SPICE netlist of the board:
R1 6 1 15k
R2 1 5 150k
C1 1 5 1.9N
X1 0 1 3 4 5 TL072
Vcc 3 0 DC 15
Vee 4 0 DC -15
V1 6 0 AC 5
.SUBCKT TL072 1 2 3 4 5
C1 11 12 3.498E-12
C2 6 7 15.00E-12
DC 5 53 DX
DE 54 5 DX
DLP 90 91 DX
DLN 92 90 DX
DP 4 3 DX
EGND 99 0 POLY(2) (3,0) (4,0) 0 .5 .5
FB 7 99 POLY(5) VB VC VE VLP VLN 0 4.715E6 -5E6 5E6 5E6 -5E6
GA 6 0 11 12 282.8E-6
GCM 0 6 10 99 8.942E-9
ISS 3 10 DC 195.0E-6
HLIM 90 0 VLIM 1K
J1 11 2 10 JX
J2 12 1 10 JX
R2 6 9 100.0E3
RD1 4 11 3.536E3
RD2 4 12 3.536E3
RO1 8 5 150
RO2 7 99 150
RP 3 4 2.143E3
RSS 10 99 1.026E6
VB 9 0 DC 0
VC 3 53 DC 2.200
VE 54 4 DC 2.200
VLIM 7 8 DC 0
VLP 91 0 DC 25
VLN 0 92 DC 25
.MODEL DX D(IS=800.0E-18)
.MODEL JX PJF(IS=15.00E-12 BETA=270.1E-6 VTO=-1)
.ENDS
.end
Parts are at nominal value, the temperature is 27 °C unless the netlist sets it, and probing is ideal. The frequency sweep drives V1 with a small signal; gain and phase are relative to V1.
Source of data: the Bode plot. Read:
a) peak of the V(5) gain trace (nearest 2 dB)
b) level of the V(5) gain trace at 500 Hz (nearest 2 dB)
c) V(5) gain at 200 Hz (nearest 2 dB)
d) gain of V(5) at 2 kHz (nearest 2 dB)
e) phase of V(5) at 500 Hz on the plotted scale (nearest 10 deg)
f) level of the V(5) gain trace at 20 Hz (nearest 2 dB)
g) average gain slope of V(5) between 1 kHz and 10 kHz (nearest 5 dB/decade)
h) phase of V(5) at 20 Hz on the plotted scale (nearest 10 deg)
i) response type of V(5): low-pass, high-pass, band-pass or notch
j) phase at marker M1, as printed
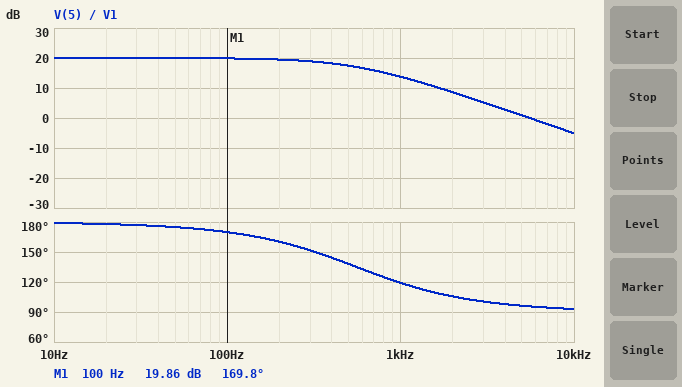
20 dB
18 dB
20 dB
8 dB
140 deg
20 dB
-20 dB/decade
180 deg
low-pass
169.8 deg
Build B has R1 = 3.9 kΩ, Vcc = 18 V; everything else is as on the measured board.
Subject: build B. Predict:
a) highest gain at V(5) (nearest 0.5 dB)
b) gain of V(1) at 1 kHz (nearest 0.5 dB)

31.5 dB
-45.5 dB
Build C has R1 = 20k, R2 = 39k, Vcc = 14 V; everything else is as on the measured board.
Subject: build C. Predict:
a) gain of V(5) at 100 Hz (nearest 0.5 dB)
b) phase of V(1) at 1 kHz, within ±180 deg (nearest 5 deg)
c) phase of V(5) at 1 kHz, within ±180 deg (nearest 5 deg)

6.0 dB
65 deg
155 deg
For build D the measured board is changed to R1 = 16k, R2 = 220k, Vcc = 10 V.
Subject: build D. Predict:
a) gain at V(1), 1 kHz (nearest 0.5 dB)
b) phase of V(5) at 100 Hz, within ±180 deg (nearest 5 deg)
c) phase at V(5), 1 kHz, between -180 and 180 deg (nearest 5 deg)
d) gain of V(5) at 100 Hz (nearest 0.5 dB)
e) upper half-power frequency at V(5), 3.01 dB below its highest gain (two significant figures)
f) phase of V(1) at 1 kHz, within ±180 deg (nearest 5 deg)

-57.0 dB
165 deg
110 deg
22.5 dB
380 Hz
20 deg
